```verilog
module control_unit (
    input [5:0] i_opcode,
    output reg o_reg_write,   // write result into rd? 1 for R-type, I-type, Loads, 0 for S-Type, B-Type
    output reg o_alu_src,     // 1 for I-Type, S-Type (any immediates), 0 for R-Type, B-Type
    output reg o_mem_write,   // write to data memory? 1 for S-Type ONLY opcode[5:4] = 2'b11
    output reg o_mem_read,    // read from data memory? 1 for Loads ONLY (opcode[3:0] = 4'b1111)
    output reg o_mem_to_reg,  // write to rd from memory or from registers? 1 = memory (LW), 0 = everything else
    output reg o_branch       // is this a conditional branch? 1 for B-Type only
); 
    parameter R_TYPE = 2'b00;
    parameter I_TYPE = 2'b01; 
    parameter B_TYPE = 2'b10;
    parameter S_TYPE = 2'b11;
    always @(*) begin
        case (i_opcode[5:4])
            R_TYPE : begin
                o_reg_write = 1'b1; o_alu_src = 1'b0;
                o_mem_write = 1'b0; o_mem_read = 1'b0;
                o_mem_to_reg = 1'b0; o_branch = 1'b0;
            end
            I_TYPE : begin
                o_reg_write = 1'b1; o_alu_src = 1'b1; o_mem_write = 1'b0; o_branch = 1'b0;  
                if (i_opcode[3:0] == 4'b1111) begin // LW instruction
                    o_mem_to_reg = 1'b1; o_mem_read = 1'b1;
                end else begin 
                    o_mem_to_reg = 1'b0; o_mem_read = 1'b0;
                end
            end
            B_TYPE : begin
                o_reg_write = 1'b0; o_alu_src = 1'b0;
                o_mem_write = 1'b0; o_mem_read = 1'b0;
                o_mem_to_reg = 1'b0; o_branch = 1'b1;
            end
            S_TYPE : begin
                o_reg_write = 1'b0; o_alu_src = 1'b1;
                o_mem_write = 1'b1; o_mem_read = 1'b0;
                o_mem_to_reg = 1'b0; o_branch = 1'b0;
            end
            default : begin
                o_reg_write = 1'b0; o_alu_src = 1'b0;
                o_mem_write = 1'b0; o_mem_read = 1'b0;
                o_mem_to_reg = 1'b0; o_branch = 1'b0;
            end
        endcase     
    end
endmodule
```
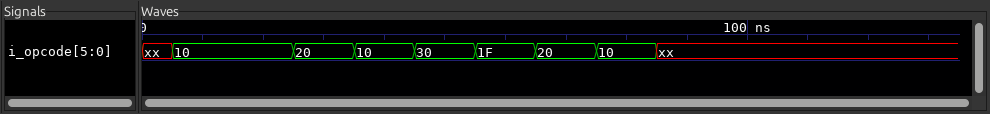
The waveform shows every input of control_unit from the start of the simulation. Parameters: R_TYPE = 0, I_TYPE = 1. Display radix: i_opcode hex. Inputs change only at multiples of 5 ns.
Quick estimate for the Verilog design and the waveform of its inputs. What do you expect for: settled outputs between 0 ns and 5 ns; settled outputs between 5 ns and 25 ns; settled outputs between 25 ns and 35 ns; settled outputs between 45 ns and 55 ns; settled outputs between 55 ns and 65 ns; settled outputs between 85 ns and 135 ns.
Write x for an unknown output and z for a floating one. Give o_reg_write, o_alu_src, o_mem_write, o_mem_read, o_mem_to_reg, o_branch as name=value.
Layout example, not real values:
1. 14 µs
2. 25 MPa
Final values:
1. o_reg_write=x, o_alu_src=x, o_mem_write=x, o_mem_read=x, o_mem_to_reg=x, o_branch=x
2. o_reg_write=1, o_alu_src=1, o_mem_write=0, o_mem_read=0, o_mem_to_reg=0, o_branch=0
3. o_reg_write=0, o_alu_src=0, o_mem_write=0, o_mem_read=0, o_mem_to_reg=0, o_branch=1
4. o_reg_write=0, o_alu_src=1, o_mem_write=1, o_mem_read=0, o_mem_to_reg=0, o_branch=0
5. o_reg_write=1, o_alu_src=1, o_mem_write=0, o_mem_read=1, o_mem_to_reg=1, o_branch=0
6. o_reg_write=0, o_alu_src=0, o_mem_write=0, o_mem_read=0, o_mem_to_reg=0, o_branch=0
